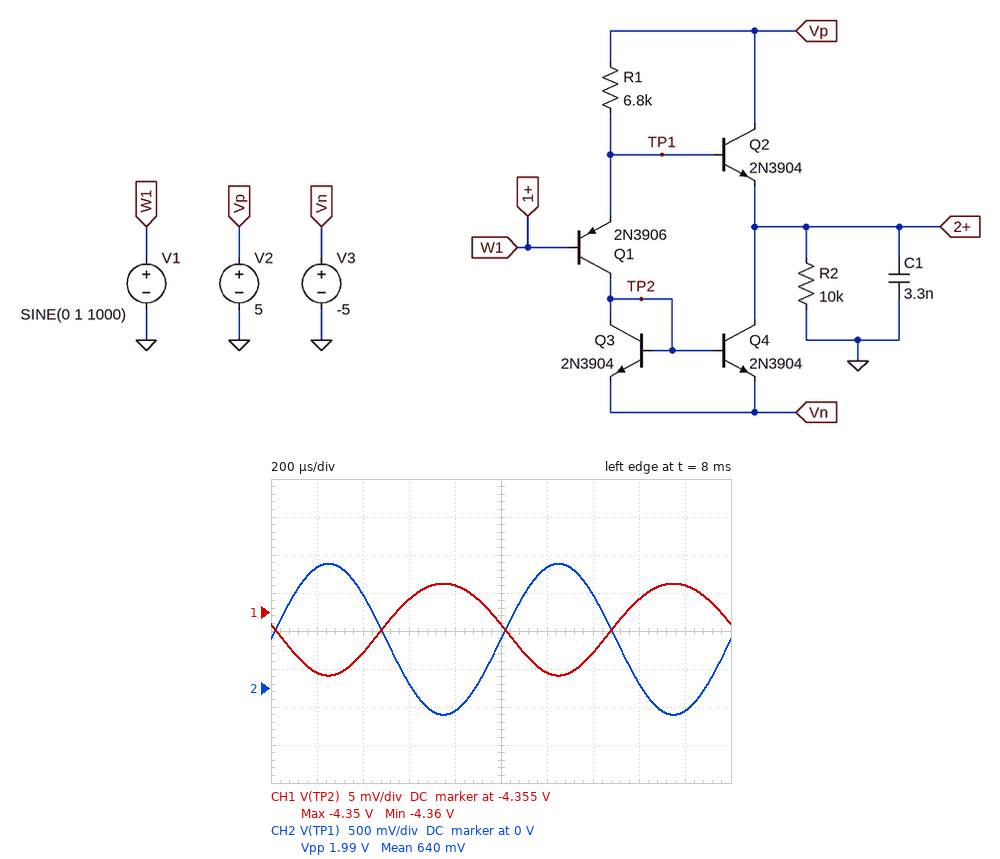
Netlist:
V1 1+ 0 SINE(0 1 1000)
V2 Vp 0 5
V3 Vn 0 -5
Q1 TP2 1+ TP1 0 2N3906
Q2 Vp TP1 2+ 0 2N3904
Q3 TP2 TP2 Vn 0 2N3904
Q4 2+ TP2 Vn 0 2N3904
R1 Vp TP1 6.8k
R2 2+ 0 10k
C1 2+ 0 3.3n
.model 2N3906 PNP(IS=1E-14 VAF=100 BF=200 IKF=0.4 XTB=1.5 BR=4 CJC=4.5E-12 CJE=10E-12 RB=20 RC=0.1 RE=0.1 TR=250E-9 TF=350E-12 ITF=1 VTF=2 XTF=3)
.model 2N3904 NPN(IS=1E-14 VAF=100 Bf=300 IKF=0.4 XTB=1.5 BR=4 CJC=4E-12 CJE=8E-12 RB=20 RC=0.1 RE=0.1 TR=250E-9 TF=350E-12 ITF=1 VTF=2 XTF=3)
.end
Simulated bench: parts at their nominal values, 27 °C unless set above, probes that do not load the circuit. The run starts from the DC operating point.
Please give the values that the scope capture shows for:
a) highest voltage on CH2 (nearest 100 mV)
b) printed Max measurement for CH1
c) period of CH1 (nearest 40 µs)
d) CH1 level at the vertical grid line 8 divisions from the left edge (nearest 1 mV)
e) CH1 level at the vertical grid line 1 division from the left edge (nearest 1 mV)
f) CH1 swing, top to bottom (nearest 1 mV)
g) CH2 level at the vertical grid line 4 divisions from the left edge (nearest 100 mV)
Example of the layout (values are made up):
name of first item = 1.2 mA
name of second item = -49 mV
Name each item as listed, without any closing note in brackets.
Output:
highest voltage on CH2 = 1.6 V
printed Max measurement for CH1 = -4.35 V
period of CH1 = 1.00 ms
CH1 level at the vertical grid line 8 divisions from the left edge = -4.353 V
CH1 level at the vertical grid line 1 division from the left edge = -4.363 V
CH1 swing, top to bottom = 12 mV
CH2 level at the vertical grid line 4 divisions from the left edge = -300 mV
